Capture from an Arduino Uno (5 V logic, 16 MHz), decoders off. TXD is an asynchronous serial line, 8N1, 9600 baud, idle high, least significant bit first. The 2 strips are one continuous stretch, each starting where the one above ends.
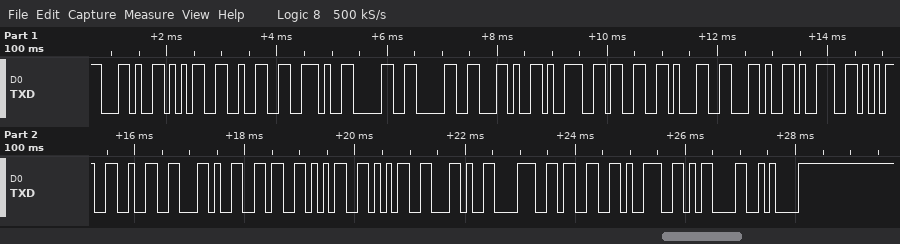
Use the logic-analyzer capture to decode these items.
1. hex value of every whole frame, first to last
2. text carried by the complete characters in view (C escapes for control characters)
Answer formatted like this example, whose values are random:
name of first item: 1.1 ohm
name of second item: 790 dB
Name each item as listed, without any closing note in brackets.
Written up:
hex value of every whole frame, first to last: 2C 35 32 2E 30 30 2C 39 33 31 2C 39 35 32 2C 36 35 35 2C 38 33 39 0D 0A
text carried by the complete characters in view: ",52.00,931,952,655,839\r\n"
